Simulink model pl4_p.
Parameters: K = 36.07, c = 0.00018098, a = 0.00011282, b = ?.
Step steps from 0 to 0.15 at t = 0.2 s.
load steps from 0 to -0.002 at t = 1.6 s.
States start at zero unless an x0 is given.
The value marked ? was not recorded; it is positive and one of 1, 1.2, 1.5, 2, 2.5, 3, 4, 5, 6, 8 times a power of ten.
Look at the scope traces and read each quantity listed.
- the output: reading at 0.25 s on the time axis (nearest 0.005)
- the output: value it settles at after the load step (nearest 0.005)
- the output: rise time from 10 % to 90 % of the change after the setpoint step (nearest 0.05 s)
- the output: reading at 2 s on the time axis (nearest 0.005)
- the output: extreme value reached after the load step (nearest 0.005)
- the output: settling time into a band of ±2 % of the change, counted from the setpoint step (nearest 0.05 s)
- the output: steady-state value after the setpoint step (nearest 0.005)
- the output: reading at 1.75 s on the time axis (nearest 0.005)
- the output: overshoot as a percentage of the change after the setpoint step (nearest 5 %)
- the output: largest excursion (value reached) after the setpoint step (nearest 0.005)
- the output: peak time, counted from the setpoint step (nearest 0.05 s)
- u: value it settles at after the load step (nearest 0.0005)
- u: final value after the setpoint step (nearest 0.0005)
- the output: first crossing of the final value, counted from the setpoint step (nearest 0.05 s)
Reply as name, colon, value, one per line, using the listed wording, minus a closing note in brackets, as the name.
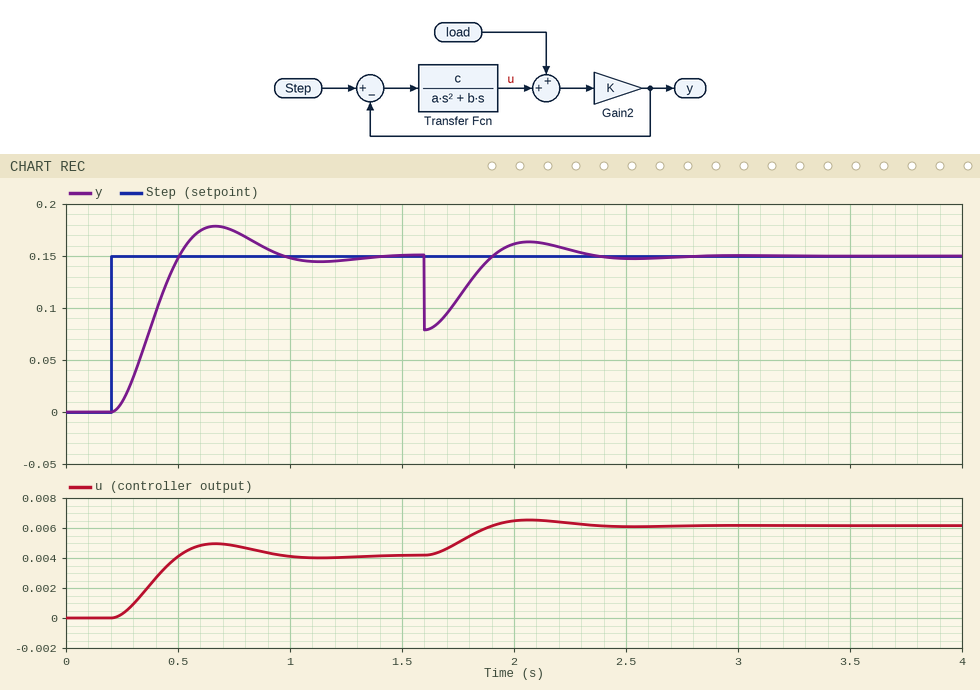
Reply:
the output: reading at 0.25 s on the time axis: 0.010
the output: value it settles at after the load step: 0.150
the output: rise time from 10 % to 90 % of the change after the setpoint step: 0.20 s
the output: reading at 2 s on the time axis: 0.160
the output: extreme value reached after the load step: 0.080
the output: settling time into a band of ±2 % of the change, counted from the setpoint step: 1.10 s
the output: steady-state value after the setpoint step: 0.150
the output: reading at 1.75 s on the time axis: 0.110
the output: overshoot as a percentage of the change after the setpoint step: 20 %
the output: largest excursion (value reached) after the setpoint step: 0.180
the output: peak time, counted from the setpoint step: 0.45 s
u: value it settles at after the load step: 0.0060
u: final value after the setpoint step: 0.0040
the output: first crossing of the final value, counted from the setpoint step: 0.30 s
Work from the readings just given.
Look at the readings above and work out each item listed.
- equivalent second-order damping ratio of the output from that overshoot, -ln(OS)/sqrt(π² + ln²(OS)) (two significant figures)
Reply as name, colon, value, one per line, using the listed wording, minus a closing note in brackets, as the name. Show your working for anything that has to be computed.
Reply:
equivalent second-order damping ratio of the output from that overshoot, -ln(OS)/sqrt(π² + ln²(OS)): ln(0.2) = -1.609; 1.609 / sqrt(9.870 + 2.590) = 0.46
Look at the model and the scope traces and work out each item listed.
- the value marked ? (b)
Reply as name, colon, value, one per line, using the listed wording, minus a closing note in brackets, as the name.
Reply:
the value marked ?: 0.0008
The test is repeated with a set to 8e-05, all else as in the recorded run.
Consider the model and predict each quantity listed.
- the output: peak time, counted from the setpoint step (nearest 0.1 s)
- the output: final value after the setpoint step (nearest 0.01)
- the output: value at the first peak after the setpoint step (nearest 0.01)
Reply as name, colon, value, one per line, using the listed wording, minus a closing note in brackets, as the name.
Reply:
the output: peak time, counted from the setpoint step: 0.4 s
the output: final value after the setpoint step: 0.15
the output: value at the first peak after the setpoint step: 0.17
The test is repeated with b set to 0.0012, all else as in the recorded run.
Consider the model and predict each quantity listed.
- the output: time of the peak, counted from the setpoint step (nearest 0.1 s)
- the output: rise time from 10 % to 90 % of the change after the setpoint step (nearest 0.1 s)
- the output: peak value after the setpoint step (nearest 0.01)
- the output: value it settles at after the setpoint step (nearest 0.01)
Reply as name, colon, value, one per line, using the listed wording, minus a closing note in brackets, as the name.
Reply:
the output: time of the peak, counted from the setpoint step: 0.6 s
the output: rise time from 10 % to 90 % of the change after the setpoint step: 0.3 s
the output: peak value after the setpoint step: 0.16
the output: value it settles at after the setpoint step: 0.15
